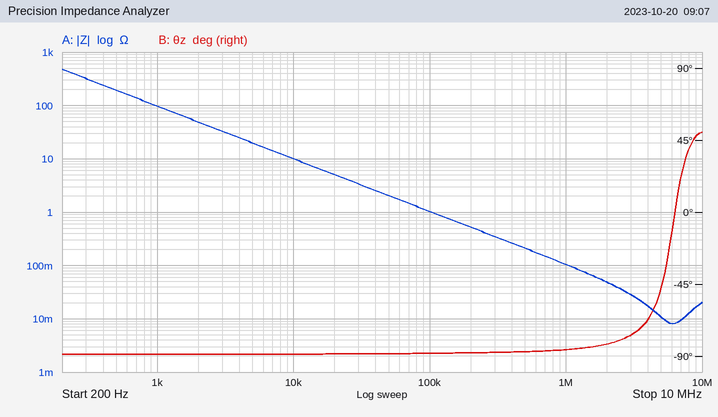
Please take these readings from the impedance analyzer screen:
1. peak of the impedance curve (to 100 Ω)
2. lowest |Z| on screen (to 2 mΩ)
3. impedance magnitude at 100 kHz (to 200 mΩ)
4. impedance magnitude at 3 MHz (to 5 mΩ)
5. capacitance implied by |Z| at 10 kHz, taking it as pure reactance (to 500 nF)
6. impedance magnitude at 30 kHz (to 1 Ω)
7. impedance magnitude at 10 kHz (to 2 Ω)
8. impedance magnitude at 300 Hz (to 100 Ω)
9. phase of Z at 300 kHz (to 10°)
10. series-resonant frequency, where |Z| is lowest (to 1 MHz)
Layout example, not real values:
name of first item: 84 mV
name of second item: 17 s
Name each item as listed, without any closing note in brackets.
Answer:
peak of the impedance curve: 500 Ω
lowest |Z| on screen: 8 mΩ
impedance magnitude at 100 kHz: 1.0 Ω
impedance magnitude at 3 MHz: 30 mΩ
capacitance implied by |Z| at 10 kHz, taking it as pure reactance: 1.5 µF
impedance magnitude at 30 kHz: 3 Ω
impedance magnitude at 10 kHz: 10 Ω
impedance magnitude at 300 Hz: 300 Ω
phase of Z at 300 kHz: -90°
series-resonant frequency, where |Z| is lowest: 6 MHz
